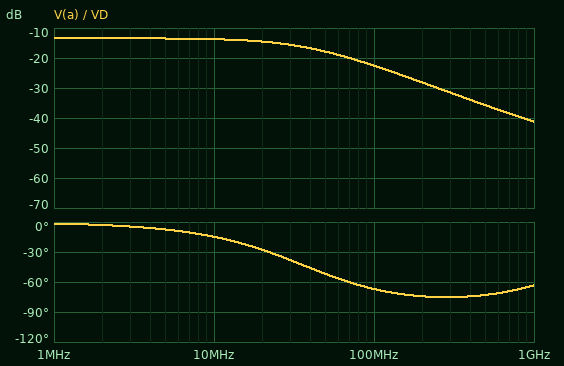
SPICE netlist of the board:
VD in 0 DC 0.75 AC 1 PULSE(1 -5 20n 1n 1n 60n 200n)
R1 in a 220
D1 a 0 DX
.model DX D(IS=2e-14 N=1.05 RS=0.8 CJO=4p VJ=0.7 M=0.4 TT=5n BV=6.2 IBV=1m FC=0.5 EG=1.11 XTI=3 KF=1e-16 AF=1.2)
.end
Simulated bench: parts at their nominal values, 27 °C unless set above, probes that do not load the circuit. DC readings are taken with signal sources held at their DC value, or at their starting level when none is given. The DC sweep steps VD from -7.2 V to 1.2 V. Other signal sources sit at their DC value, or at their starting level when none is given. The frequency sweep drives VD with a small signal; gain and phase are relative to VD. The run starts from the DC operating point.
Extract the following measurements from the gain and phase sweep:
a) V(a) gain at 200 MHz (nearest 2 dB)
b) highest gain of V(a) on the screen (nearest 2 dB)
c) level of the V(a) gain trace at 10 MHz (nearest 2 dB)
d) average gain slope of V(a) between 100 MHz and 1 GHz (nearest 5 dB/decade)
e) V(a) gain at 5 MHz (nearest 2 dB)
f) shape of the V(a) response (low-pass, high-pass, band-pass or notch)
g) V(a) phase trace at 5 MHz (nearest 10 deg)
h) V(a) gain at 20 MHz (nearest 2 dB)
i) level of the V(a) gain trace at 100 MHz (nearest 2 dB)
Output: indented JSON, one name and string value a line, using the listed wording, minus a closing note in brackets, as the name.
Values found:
{
  "V(a) gain at 200 MHz": "-28 dB",
  "highest gain of V(a) on the screen": "-14 dB",
  "level of the V(a) gain trace at 10 MHz": "-14 dB",
  "average gain slope of V(a) between 100 MHz and 1 GHz": "-20 dB/decade",
  "V(a) gain at 5 MHz": "-14 dB",
  "shape of the V(a) response": "low-pass",
  "V(a) phase trace at 5 MHz": "-10 deg",
  "V(a) gain at 20 MHz": "-14 dB",
  "level of the V(a) gain trace at 100 MHz": "-22 dB"
}
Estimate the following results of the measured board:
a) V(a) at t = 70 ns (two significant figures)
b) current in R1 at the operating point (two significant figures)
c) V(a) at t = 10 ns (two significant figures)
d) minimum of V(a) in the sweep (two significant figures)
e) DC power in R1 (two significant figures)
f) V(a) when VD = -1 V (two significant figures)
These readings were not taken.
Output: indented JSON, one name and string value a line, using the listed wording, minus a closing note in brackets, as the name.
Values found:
{
  "V(a) at t = 70 ns": "-5.0 V",
  "current in R1 at the operating point": "460 µA",
  "V(a) at t = 10 ns": "680 mV",
  "minimum of V(a) in the sweep": "-6.2 V",
  "DC power in R1": "47 µW",
  "V(a) when VD = -1 V": "-1.0 V"
}
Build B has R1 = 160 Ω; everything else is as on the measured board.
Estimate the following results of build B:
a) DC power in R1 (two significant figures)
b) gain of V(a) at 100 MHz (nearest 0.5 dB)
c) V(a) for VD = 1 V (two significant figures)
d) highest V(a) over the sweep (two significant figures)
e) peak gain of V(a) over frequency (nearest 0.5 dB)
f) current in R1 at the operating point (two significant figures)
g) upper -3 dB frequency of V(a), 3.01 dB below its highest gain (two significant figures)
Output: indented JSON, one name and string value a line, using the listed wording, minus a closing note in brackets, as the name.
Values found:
{
  "DC power in R1": "56 µW",
  "gain of V(a) at 100 MHz": "-22.0 dB",
  "V(a) for VD = 1 V": "690 mV",
  "highest V(a) over the sweep": "700 mV",
  "peak gain of V(a) over frequency": "-13.0 dB",
  "current in R1 at the operating point": "590 µA",
  "upper -3 dB frequency of V(a), 3.01 dB below its highest gain": "38 MHz"
}
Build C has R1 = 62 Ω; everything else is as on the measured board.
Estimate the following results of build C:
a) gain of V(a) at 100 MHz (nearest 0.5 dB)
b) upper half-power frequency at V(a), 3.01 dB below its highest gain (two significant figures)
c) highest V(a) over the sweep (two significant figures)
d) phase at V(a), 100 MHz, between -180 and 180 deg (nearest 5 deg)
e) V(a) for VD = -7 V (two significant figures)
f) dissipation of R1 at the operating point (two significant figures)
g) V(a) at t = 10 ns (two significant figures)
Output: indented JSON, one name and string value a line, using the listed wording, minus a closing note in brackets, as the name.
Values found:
{
  "gain of V(a) at 100 MHz": "-19.5 dB",
  "upper half-power frequency at V(a), 3.01 dB below its highest gain": "42 MHz",
  "highest V(a) over the sweep": "730 mV",
  "phase at V(a), 100 MHz, between -180 and 180 deg": "-60 deg",
  "V(a) for VD = -7 V": "-6.3 V",
  "dissipation of R1 at the operating point": "90 µW",
  "V(a) at t = 10 ns": "710 mV"
}
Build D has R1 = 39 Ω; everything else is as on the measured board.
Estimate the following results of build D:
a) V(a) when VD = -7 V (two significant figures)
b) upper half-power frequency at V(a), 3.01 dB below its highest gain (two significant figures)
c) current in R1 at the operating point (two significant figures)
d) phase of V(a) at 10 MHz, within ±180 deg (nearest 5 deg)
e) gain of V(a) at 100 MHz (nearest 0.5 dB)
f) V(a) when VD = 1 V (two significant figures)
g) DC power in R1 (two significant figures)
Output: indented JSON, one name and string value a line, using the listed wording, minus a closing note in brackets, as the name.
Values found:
{
  "V(a) when VD = -7 V": "-6.3 V",
  "upper half-power frequency at V(a), 3.01 dB below its highest gain": "44 MHz",
  "current in R1 at the operating point": "1.7 mA",
  "phase of V(a) at 10 MHz, within ±180 deg": "-10 deg",
  "gain of V(a) at 100 MHz": "-18.0 dB",
  "V(a) when VD = 1 V": "730 mV",
  "DC power in R1": "110 µW"
}
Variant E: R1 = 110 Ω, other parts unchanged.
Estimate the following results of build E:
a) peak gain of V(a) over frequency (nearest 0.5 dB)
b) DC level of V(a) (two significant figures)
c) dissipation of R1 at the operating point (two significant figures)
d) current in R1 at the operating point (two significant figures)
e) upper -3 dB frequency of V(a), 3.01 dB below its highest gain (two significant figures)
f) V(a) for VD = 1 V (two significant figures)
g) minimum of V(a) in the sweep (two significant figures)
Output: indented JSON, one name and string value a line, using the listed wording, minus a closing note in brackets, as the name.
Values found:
{
  "peak gain of V(a) over frequency": "-12.5 dB",
  "DC level of V(a)": "660 mV",
  "dissipation of R1 at the operating point": "68 µW",
  "current in R1 at the operating point": "790 µA",
  "upper -3 dB frequency of V(a), 3.01 dB below its highest gain": "40 MHz",
  "V(a) for VD = 1 V": "700 mV",
  "minimum of V(a) in the sweep": "-6.3 V"
}
